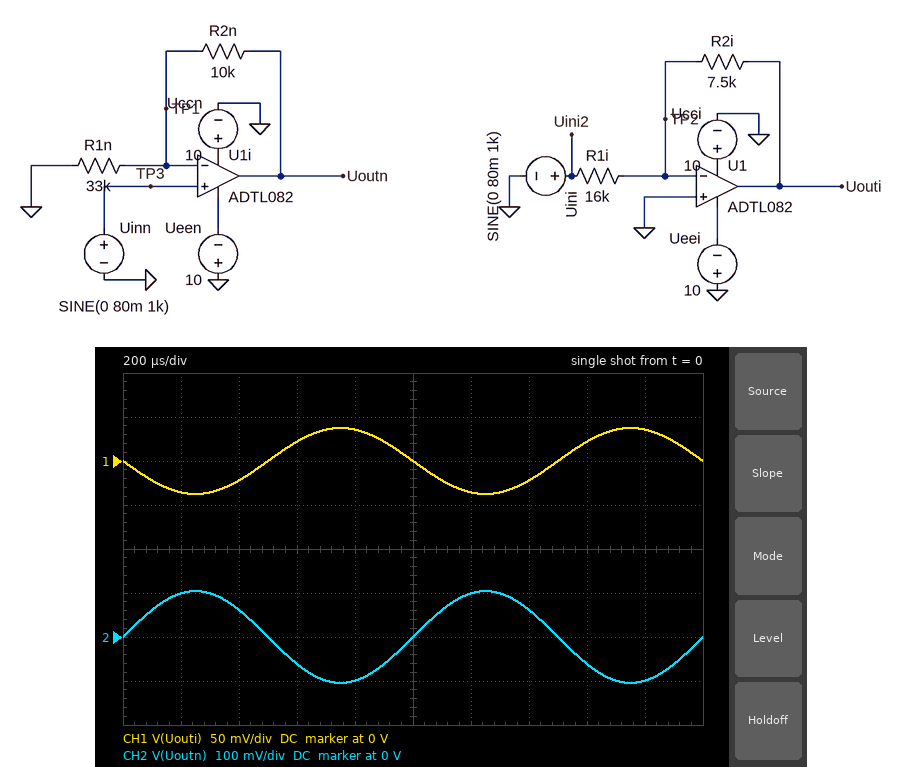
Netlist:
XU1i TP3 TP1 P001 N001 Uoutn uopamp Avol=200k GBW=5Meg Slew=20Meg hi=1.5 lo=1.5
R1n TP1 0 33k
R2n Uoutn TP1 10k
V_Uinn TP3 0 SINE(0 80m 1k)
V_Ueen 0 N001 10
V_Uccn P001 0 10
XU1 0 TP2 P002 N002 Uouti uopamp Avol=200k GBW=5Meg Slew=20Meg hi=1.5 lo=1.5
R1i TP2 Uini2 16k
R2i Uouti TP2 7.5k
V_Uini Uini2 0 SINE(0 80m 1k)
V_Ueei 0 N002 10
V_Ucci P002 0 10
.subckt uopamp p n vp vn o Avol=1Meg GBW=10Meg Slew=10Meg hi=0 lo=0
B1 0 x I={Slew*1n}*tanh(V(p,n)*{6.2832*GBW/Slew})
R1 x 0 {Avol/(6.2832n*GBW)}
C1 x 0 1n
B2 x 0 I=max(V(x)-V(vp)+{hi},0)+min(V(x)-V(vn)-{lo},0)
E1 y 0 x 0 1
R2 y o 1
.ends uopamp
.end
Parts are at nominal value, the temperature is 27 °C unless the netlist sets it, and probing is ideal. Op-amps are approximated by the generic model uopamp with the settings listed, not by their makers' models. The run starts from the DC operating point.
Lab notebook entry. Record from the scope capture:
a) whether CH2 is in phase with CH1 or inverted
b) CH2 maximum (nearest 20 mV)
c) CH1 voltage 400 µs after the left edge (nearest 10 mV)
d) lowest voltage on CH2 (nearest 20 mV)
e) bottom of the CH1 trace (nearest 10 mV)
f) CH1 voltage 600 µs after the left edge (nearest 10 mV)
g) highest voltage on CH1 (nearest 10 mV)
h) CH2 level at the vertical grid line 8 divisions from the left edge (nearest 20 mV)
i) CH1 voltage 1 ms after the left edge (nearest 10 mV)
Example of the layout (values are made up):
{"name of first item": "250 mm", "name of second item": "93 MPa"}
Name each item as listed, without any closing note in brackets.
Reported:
{"whether CH2 is in phase with CH1 or inverted": "inverted", "CH2 maximum": "100 mV", "CH1 voltage 400 µs after the left edge": "-20 mV", "lowest voltage on CH2": "-100 mV", "bottom of the CH1 trace": "-40 mV", "CH1 voltage 600 µs after the left edge": "20 mV", "highest voltage on CH1": "40 mV", "CH2 level at the vertical grid line 8 divisions from the left edge": "-60 mV", "CH1 voltage 1 ms after the left edge": "0 V"}
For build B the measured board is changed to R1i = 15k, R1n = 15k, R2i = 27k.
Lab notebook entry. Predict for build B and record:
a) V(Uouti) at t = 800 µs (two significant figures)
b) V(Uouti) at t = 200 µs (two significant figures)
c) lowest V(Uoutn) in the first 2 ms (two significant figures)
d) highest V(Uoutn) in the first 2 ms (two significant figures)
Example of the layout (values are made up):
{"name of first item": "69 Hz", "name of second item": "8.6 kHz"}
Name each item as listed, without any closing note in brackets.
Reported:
{"V(Uouti) at t = 800 µs": "140 mV", "V(Uouti) at t = 200 µs": "-140 mV", "lowest V(Uoutn) in the first 2 ms": "-130 mV", "highest V(Uoutn) in the first 2 ms": "130 mV"}
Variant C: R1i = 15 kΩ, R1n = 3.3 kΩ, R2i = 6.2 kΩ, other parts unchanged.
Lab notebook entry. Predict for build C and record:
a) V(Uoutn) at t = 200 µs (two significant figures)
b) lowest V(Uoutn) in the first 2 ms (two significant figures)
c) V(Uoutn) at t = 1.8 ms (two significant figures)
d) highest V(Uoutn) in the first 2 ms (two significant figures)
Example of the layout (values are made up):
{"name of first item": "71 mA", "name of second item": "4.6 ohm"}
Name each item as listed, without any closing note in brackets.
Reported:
{"V(Uoutn) at t = 200 µs": "310 mV", "lowest V(Uoutn) in the first 2 ms": "-320 mV", "V(Uoutn) at t = 1.8 ms": "-310 mV", "highest V(Uoutn) in the first 2 ms": "320 mV"}
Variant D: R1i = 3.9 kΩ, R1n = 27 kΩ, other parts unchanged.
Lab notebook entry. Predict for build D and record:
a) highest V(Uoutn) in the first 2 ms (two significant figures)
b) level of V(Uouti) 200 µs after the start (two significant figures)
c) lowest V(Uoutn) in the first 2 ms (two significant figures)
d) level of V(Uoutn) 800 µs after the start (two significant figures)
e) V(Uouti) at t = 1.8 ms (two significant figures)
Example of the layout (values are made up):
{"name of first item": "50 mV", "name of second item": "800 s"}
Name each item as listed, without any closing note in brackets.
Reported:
{"highest V(Uoutn) in the first 2 ms": "110 mV", "level of V(Uouti) 200 µs after the start": "-150 mV", "lowest V(Uoutn) in the first 2 ms": "-110 mV", "level of V(Uoutn) 800 µs after the start": "-100 mV", "V(Uouti) at t = 1.8 ms": "150 mV"}
